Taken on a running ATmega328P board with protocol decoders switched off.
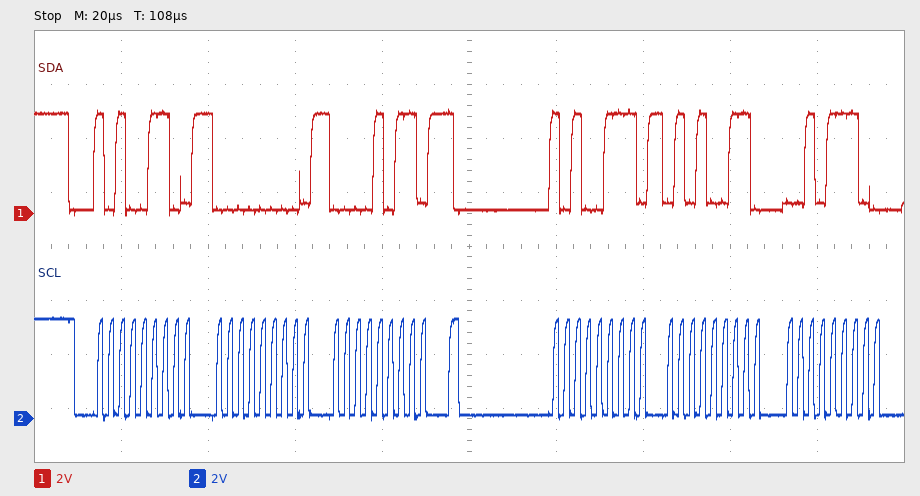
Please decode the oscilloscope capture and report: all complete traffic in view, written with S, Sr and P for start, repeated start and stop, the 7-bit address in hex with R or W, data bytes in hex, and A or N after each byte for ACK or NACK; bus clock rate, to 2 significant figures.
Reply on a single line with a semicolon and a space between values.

S 53W A 00 A 0B A Sr 53R A 53 A 2E A; 400 kHz
